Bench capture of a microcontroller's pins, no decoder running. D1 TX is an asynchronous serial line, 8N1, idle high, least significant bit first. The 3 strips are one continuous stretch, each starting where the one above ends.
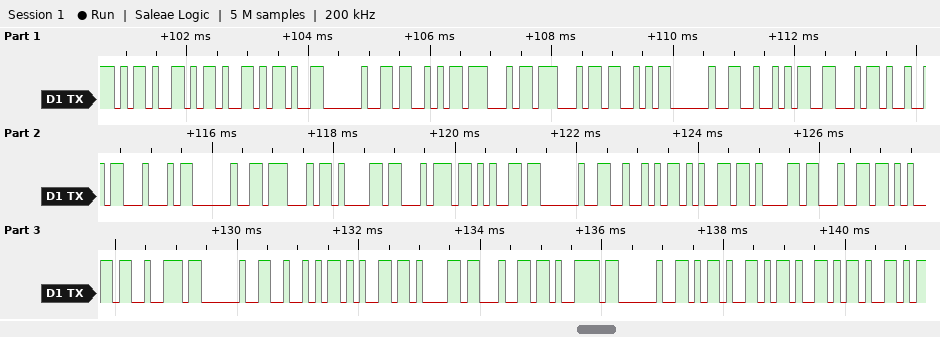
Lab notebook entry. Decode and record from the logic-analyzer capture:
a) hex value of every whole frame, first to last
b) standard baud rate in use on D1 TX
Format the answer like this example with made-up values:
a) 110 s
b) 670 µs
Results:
a) 2D 2D 2D 20 53 47 47 53 20 52 46 49 44 20 47 61 74 65 20 52 65 61 64 65 72 20 52 65 61 64 79 20 2D 2D 2D
b) 9600 baud
